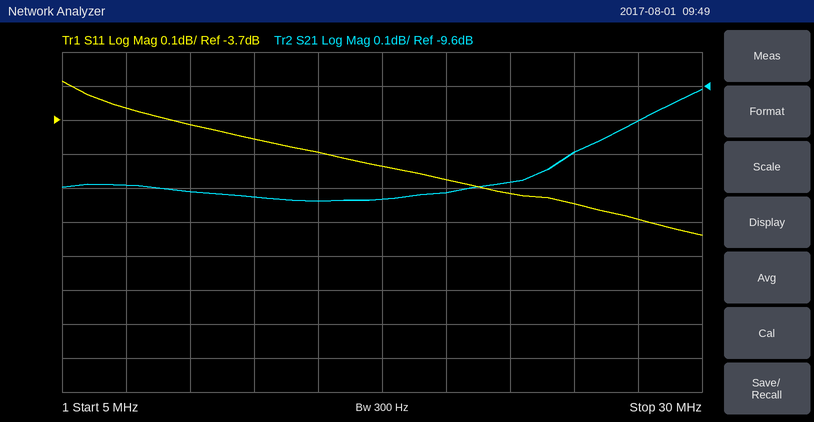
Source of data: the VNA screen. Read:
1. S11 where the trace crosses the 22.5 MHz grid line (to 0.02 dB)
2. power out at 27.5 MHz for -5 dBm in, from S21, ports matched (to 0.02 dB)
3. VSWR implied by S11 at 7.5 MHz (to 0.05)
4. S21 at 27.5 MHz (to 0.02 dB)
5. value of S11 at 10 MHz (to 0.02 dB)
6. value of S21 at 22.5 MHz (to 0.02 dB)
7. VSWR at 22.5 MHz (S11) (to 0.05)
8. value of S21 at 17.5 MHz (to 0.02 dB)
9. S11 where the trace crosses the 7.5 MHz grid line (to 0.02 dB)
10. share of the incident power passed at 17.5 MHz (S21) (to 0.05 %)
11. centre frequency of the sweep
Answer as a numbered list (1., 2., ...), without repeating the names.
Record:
1. -3.92 dB
2. -14.70 dBm
3. 4.80
4. -9.70 dB
5. -3.72 dB
6. -9.88 dB
7. 4.50
8. -9.94 dB
9. -3.66 dB
10. 10.15 %
11. 17.5 MHz
